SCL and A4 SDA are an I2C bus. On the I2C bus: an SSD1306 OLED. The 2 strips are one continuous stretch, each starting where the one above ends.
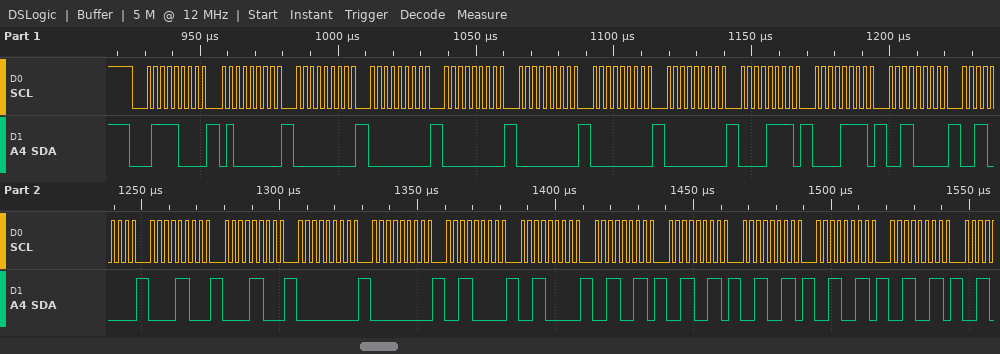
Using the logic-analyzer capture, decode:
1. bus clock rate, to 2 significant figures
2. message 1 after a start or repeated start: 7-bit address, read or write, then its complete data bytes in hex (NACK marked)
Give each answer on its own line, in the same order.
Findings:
400 kHz
0x3C write: 40 00 00 00 00 00 00 0F 0F 30 30 0C 0C 00 00 30 30 33 33 33 33 33
